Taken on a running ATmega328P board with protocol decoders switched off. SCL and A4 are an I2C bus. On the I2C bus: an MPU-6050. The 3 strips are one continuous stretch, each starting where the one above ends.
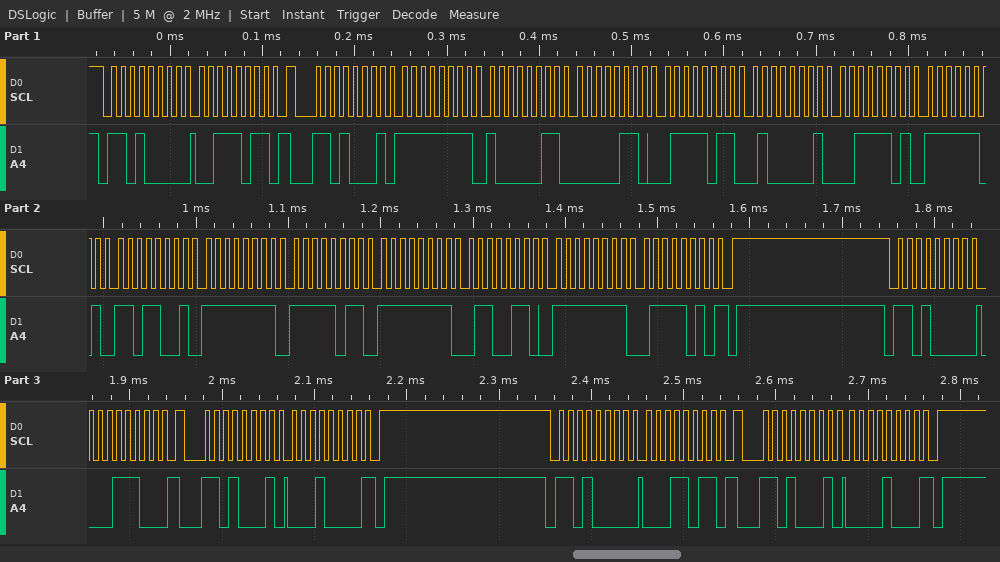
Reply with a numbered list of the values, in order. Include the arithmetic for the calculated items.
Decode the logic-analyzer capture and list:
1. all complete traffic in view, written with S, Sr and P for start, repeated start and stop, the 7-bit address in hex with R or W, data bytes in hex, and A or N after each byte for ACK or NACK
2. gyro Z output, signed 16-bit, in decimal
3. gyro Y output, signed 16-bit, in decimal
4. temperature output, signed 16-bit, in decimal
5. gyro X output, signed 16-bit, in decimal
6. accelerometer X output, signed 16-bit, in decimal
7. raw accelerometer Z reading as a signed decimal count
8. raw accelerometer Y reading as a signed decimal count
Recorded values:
1. S 68W A 3B A Sr 68R A FF A 83 A 06 A 7B A 41 A 3D A FD A D9 A FF A FB A FF A 66 A FF A 7A N P S 68W A 1C A Sr 68R A 10 N P S 68W A 1B A Sr 68R A 08 N P
2. 0xFF7A = -134
3. 0xFF66 = -154
4. 0xFDD9 = -551
5. 0xFFFB = -5
6. 0xFF83 = -125
7. 0x413D = 16701
8. 0x067B = 1659
